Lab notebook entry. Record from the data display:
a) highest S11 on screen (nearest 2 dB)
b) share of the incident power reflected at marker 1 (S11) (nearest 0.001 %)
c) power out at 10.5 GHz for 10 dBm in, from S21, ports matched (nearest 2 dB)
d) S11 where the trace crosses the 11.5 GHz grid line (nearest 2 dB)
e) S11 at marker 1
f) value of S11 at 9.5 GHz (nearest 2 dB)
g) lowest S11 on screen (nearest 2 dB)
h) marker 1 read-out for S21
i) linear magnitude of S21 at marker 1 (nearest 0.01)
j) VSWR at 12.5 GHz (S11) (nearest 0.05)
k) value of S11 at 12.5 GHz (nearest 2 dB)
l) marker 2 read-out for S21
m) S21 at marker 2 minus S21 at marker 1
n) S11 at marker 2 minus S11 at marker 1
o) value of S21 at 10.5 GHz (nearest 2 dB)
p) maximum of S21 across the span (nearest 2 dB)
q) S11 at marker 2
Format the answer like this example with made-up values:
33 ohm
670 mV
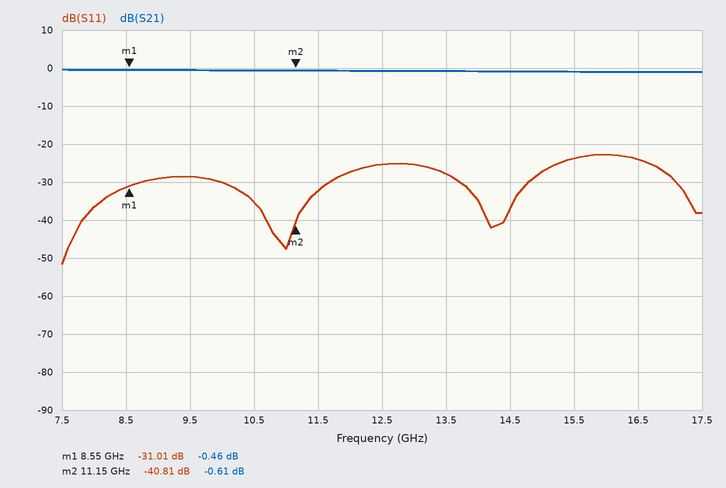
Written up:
-22 dB
0.079 %
10 dBm
-32 dB
-31.01 dB
-28 dB
-52 dB
-0.46 dB
0.95
1.10
-26 dB
-0.61 dB
-0.15 dB
-9.80 dB
0 dB
0 dB
-40.81 dB
